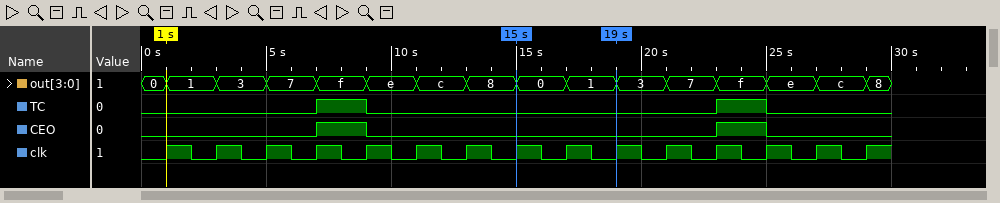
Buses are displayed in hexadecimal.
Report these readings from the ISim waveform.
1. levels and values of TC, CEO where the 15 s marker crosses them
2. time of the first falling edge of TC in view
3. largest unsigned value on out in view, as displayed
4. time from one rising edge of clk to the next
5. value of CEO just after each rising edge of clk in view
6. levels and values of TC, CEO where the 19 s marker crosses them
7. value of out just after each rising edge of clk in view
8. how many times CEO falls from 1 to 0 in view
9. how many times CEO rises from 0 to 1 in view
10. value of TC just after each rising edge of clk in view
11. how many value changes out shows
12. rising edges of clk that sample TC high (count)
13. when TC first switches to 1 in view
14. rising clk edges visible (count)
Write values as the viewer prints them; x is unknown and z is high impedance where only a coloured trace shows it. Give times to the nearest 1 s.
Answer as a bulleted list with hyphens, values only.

- TC=0, CEO=0
- 9 s
- f
- 2 s
- 0 0 0 1 0 0 0 0 0 0 0 1 0 0 0
- TC=0, CEO=0
- 1, 3, 7, f, e, c, 8, 0, 1, 3, 7, f, e, c, 8
- 2
- 2
- 0 0 0 1 0 0 0 0 0 0 0 1 0 0 0
- 15
- 2
- 7 s
- 15
